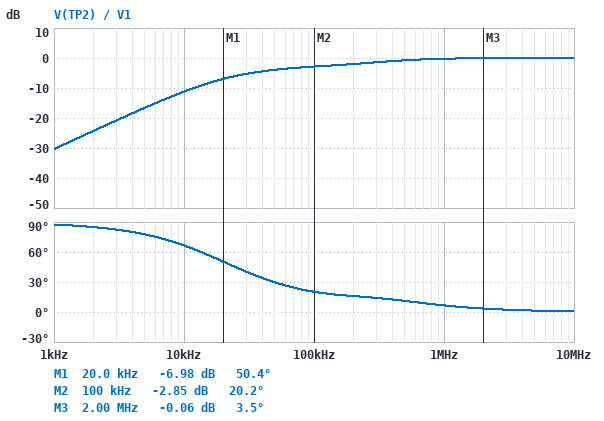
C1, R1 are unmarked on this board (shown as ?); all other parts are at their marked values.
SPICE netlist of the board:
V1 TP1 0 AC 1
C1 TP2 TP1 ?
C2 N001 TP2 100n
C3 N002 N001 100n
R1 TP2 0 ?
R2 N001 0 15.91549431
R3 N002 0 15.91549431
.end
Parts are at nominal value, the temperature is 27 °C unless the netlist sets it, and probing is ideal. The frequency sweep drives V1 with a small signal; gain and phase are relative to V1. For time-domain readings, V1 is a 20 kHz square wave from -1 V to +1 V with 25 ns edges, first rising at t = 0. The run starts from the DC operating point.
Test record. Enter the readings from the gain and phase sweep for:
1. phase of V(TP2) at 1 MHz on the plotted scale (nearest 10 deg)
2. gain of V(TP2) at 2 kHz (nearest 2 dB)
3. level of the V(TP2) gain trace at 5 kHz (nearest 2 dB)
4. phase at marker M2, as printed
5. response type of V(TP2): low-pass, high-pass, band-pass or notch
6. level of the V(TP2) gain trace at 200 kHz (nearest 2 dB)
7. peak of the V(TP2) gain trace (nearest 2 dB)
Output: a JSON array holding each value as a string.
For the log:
["10 deg", "-24 dB", "-16 dB", "20.2 deg", "high-pass", "-2 dB", "0 dB"]
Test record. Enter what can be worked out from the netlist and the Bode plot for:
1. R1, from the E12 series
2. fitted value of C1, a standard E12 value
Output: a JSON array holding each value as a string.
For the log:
["22 Ω", "220 nF"]
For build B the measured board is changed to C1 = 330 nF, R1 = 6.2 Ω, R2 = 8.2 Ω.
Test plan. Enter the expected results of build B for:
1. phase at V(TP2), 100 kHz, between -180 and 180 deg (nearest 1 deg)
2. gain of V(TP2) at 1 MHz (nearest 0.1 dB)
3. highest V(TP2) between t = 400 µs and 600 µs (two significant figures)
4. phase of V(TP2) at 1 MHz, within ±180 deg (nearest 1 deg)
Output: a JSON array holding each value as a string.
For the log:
["35 deg", "-0.3 dB", "2.0 V", "9 deg"]
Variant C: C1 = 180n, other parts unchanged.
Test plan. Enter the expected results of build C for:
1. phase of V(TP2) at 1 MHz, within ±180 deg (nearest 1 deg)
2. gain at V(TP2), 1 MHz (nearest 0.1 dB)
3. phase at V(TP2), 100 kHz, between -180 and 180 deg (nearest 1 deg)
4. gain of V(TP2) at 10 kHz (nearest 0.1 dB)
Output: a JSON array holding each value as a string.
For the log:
["8 deg", "-0.3 dB", "23 deg", "-12.8 dB"]
